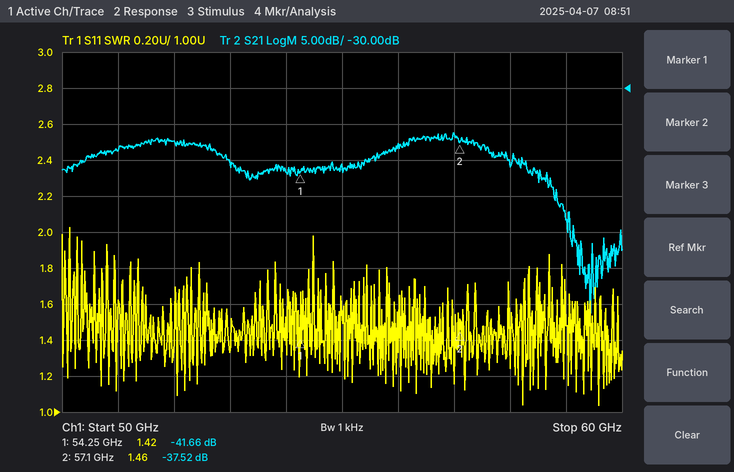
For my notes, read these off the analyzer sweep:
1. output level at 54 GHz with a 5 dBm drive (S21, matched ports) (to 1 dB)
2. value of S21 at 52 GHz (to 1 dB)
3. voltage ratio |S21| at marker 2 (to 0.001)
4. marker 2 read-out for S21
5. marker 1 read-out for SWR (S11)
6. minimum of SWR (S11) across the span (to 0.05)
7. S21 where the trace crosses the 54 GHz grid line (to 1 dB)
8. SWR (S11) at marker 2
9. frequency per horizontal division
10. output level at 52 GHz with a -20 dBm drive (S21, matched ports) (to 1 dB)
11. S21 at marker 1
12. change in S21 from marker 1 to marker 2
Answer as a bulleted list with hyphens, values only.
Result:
- -37 dBm
- -37 dB
- 0.013
- -37.52 dB
- 1.42
- 1.05
- -42 dB
- 1.46
- 1 GHz
- -57 dBm
- -41.66 dB
- 4.14 dB
